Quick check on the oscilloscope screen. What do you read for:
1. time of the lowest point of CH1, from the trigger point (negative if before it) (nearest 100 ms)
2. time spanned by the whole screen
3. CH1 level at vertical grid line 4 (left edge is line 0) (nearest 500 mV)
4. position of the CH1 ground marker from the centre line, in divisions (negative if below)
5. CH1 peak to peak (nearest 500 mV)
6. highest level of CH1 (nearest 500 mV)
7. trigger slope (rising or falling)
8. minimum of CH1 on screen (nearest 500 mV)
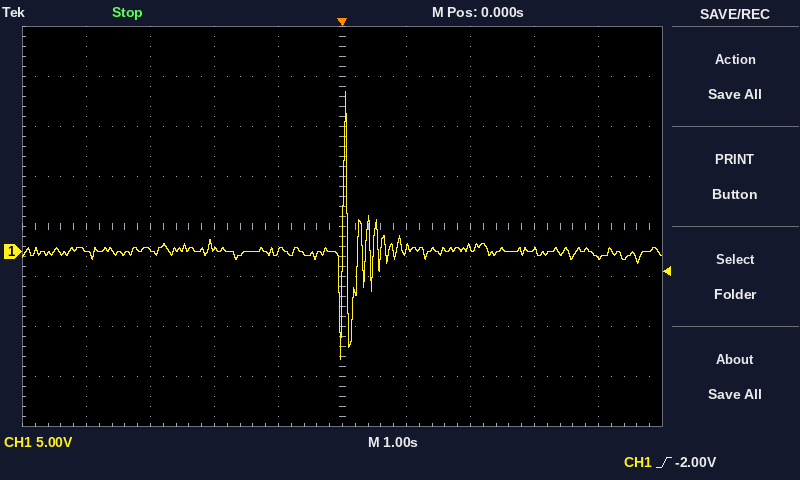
0.0 s
10 s
0.0 V
-0.5 div
27.0 V
16.0 V
rising
-11.0 V
